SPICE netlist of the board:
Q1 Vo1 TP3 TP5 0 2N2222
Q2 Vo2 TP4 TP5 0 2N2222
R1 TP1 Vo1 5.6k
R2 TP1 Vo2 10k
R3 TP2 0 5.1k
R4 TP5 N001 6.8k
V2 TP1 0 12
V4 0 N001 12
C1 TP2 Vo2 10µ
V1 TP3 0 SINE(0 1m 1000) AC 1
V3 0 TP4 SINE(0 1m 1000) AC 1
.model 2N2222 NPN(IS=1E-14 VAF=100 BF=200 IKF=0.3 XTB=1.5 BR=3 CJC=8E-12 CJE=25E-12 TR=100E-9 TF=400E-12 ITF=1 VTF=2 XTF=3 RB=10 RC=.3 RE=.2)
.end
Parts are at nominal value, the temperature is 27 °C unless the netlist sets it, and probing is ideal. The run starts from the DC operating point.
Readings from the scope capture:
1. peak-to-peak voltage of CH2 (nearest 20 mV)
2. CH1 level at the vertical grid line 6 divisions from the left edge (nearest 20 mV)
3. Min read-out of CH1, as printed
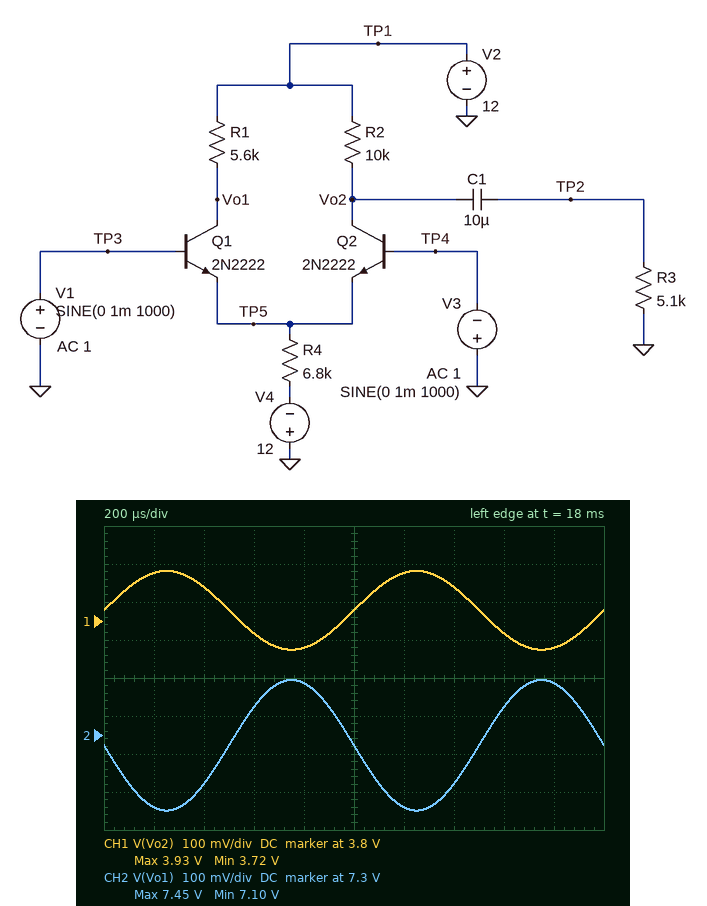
340 mV
3.92 V
3.72 V
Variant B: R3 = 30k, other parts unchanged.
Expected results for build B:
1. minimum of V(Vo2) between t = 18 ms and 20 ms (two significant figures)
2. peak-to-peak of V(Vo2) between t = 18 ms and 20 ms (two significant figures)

3.6 V
450 mV
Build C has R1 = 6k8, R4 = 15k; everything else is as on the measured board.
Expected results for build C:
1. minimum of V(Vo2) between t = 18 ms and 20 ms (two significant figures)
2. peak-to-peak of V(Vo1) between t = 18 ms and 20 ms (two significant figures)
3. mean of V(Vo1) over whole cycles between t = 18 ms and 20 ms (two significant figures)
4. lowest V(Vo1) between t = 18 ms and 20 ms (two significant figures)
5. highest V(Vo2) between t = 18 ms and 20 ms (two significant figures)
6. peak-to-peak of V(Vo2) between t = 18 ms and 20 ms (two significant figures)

8.2 V
190 mV
9.4 V
9.3 V
8.3 V
96 mV
